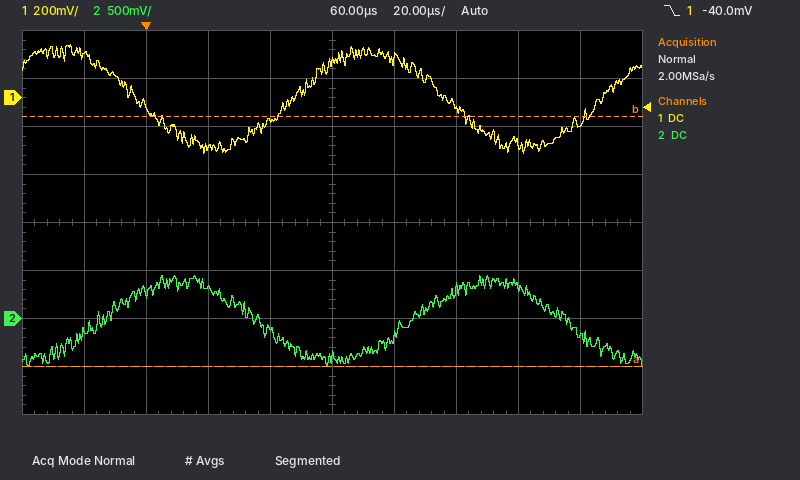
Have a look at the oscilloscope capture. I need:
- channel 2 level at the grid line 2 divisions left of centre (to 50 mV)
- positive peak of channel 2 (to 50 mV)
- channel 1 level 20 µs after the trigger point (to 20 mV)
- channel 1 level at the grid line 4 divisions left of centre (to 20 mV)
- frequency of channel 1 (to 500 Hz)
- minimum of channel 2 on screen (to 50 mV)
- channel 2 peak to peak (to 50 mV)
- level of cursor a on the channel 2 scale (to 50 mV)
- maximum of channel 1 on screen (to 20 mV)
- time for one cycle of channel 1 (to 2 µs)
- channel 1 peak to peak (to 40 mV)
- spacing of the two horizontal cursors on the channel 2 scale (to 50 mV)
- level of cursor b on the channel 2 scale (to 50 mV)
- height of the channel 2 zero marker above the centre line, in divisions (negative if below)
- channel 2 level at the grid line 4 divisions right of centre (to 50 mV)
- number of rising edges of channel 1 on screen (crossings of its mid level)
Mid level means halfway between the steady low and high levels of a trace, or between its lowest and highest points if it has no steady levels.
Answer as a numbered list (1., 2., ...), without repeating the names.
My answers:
1. 300 mV
2. 450 mV
3. -200 mV
4. 180 mV
5. 10.0 kHz
6. -500 mV
7. 950 mV
8. -500 mV
9. 220 mV
10. 100 µs
11. 440 mV
12. 2.60 V
13. 2.10 V
14. -2.0 div
15. -200 mV
16. 2
